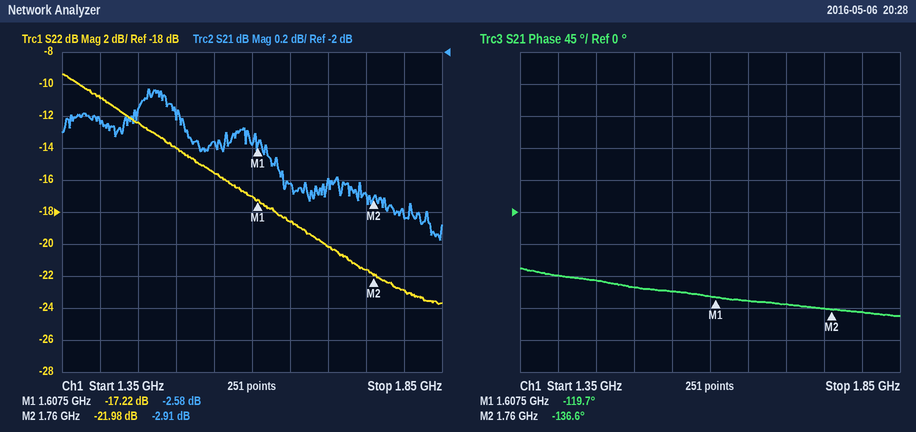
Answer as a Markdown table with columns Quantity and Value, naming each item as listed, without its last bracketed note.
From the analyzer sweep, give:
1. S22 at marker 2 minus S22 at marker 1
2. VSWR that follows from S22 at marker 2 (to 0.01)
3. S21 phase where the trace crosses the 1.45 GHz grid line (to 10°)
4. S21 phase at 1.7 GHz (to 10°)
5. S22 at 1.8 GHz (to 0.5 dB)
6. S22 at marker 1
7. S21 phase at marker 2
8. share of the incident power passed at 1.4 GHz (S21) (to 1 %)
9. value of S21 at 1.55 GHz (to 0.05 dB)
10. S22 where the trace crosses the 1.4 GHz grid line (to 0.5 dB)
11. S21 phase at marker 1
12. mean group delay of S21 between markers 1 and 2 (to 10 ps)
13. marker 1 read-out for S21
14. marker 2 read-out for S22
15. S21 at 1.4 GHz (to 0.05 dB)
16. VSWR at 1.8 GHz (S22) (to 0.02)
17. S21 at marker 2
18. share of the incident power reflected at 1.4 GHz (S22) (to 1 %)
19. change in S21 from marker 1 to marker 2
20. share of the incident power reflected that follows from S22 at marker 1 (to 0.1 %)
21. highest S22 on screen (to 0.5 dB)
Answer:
| Quantity | Value |
|---|---|
| S22 at marker 2 minus S22 at marker 1 | -4.76 dB |
| VSWR that follows from S22 at marker 2 | 1.17 |
| S21 phase where the trace crosses the 1.45 GHz grid line | -100° |
| S21 phase at 1.7 GHz | -130° |
| S22 at 1.8 GHz | -23.0 dB |
| S22 at marker 1 | -17.22 dB |
| S21 phase at marker 2 | -136.6° |
| share of the incident power passed at 1.4 GHz (S21) | 57 % |
| value of S21 at 1.55 GHz | -2.55 dB |
| S22 where the trace crosses the 1.4 GHz grid line | -11.0 dB |
| S21 phase at marker 1 | -119.7° |
| mean group delay of S21 between markers 1 and 2 | 310 ps |
| marker 1 read-out for S21 | -2.58 dB |
| marker 2 read-out for S22 | -21.98 dB |
| S21 at 1.4 GHz | -2.45 dB |
| VSWR at 1.8 GHz (S22) | 1.16 |
| S21 at marker 2 | -2.91 dB |
| share of the incident power reflected at 1.4 GHz (S22) | 8 % |
| change in S21 from marker 1 to marker 2 | -0.33 dB |
| share of the incident power reflected that follows from S22 at marker 1 | 1.9 % |
| highest S22 on screen | -9.5 dB |
